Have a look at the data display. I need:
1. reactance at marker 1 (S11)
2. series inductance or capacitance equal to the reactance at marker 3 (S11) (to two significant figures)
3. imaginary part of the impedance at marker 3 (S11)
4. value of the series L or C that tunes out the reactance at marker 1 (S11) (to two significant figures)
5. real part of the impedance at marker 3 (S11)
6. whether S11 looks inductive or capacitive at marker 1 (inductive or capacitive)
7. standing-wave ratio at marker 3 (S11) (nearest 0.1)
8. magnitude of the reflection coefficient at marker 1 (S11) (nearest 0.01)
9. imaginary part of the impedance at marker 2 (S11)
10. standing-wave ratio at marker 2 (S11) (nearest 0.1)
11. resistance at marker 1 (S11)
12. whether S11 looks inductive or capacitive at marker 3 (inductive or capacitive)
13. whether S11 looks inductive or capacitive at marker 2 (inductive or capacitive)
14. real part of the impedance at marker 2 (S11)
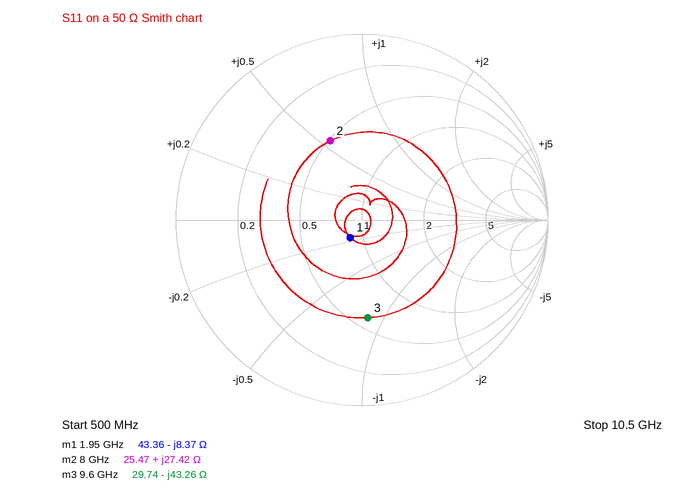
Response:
-8.37 Ω
380 fF
-43.26 Ω
680 pH
29.74 Ω
capacitive
3.2
0.11
+27.42 Ω
2.7
43.36 Ω
capacitive
inductive
25.47 Ω
